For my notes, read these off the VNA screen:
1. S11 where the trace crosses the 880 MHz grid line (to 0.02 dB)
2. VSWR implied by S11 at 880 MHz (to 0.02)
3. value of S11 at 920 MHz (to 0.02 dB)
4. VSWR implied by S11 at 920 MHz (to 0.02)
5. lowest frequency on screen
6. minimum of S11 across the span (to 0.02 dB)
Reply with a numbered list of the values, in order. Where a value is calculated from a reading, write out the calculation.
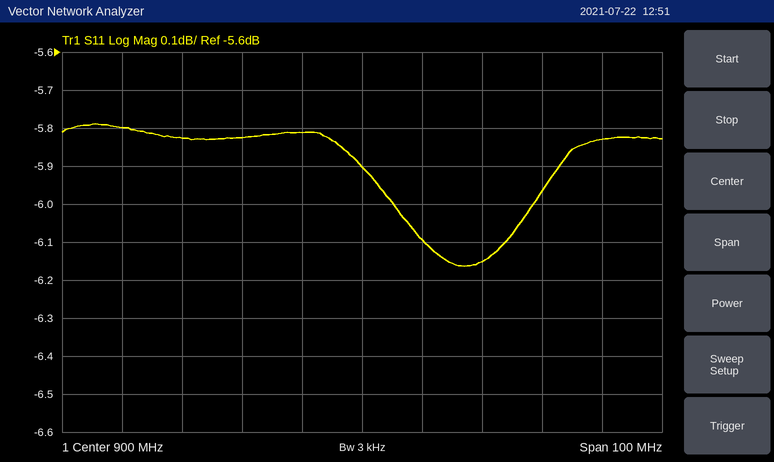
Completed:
1. -5.82 dB
2. |Γ| = 10^(-5.82/20) = 0.5117; VSWR = (1 + 0.5117)/(1 − 0.5117) ≈ 3.10
3. -6.16 dB
4. |Γ| = 10^(-6.16/20) = 0.4920; VSWR = (1 + 0.4920)/(1 − 0.4920) ≈ 2.94
5. 850 MHz
6. -6.16 dB
